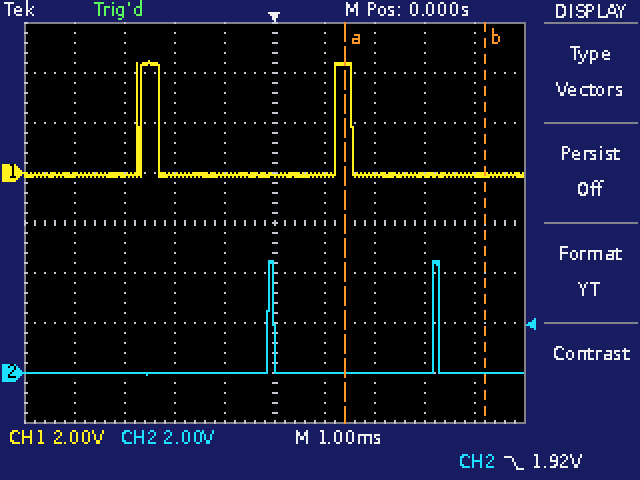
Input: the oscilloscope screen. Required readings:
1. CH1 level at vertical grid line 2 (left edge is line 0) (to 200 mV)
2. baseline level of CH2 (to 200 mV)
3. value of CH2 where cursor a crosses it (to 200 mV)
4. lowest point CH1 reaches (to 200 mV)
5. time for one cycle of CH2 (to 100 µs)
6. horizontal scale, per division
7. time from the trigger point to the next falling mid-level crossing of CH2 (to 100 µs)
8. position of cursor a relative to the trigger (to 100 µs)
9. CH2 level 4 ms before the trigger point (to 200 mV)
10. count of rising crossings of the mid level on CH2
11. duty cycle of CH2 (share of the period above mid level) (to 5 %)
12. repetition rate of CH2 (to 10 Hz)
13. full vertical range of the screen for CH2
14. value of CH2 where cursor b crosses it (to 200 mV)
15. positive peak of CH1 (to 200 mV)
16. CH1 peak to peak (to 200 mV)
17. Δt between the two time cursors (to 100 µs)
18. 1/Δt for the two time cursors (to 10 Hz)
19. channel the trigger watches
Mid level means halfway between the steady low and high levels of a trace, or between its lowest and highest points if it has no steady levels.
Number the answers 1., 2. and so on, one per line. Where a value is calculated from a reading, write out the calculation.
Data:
1. 0.0 V
2. 0.0 V
3. 0.0 V
4. -200 mV
5. 3.3 ms
6. 1 ms
7. 3.3 ms
8. +1.4 ms
9. 0.0 V
10. 2
11. 5 %
12. 1 / 3.3 ms ≈ 303 Hz, so 300 Hz to the nearest 10 Hz
13. 16 V
14. 0.0 V
15. 4.4 V
16. 4.4 V − (-200 mV) = 4.6 V
17. 2.8 ms
18. 1 / 2.8 ms ≈ 360 Hz
19. CH2
